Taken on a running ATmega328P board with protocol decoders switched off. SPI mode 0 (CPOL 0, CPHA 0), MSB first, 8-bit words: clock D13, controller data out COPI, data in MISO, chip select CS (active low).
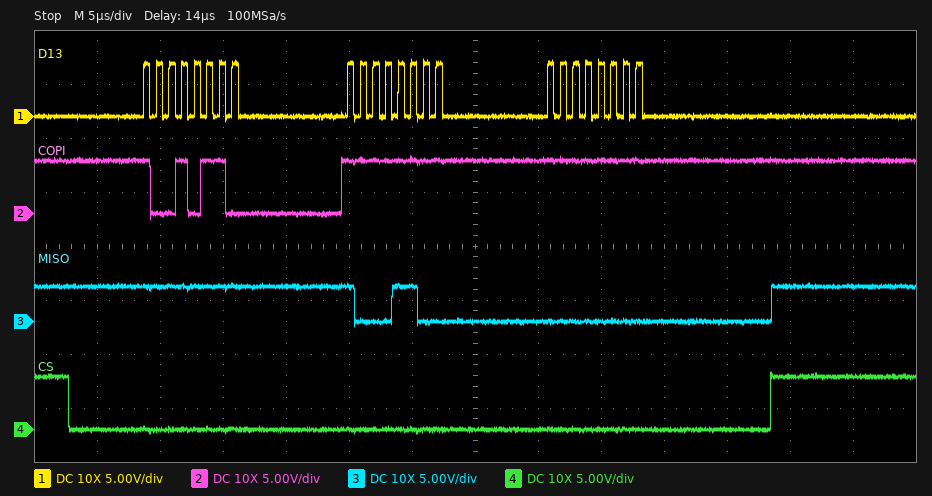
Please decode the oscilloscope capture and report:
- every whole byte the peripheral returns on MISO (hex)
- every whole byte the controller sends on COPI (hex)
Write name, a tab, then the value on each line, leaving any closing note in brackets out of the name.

every whole byte the peripheral returns on MISO	0xFF 0x8C 0x00
every whole byte the controller sends on COPI	0x96 0xFF 0xFF
